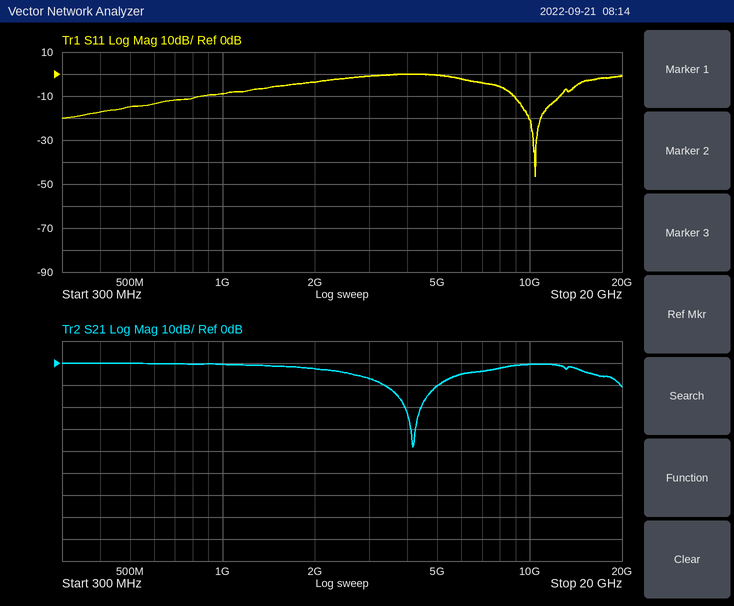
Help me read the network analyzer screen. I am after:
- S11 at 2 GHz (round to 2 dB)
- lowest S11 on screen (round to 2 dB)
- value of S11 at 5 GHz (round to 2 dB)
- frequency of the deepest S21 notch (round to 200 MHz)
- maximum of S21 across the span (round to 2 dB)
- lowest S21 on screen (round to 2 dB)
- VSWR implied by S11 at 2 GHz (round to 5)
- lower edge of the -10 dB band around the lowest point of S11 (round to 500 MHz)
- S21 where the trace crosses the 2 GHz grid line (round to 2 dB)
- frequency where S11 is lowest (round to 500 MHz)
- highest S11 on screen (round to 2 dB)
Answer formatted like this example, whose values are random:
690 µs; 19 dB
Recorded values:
-4 dB; -46 dB; 0 dB; 4.2 GHz; 0 dB; -38 dB; 5; 9.0 GHz; -2 dB; 10.5 GHz; 0 dB
